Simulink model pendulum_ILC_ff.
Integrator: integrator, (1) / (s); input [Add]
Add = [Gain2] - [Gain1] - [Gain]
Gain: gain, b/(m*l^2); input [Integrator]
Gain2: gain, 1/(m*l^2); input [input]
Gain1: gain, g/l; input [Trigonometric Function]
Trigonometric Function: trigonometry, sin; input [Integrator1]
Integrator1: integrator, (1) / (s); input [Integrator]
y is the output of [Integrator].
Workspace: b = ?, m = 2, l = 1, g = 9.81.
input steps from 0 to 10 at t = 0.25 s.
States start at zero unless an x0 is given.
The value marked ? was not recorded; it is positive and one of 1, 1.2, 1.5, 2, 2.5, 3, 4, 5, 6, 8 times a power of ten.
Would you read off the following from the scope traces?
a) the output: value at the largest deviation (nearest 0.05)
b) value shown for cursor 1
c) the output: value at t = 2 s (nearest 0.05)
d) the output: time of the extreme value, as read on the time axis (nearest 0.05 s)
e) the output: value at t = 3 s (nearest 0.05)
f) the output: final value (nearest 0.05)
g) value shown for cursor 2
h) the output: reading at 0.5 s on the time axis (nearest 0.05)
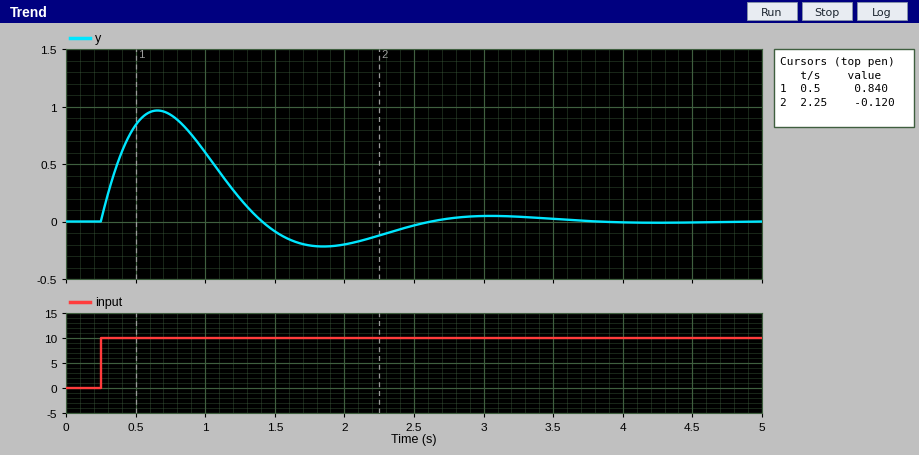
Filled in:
0.95
0.840
-0.20
0.65 s
0.05
0.00
-0.120
0.85
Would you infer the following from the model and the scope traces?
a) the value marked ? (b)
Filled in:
5
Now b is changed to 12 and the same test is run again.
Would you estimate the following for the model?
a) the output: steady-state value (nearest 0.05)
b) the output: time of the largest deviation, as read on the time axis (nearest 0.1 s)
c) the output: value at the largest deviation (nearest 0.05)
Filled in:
0.00
0.6 s
0.60
